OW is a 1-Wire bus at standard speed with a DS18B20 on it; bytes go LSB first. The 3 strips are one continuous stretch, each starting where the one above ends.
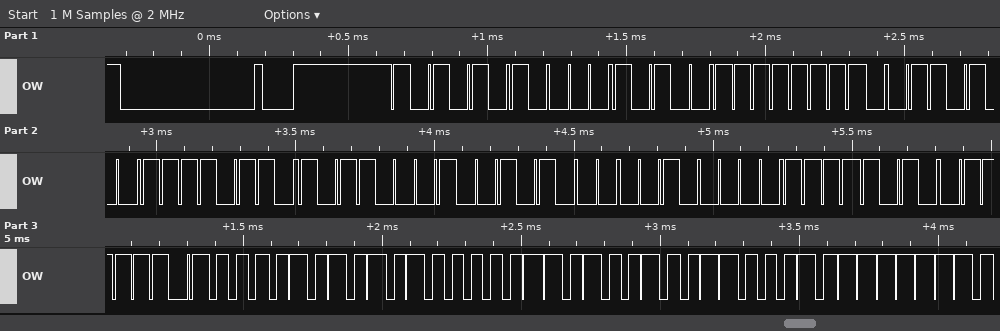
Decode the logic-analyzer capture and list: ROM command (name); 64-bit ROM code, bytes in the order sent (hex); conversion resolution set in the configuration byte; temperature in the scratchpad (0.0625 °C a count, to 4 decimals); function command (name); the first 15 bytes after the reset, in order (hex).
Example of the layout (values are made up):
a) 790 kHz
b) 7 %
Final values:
a) Match ROM
b) 28 FF 2C 6F 8D 14 04 5F
c) 12 bits
d) 85.0000 °C
e) Read Scratchpad
f) 55 28 FF 2C 6F 8D 14 04 5F BE 50 05 4B 46 7F
